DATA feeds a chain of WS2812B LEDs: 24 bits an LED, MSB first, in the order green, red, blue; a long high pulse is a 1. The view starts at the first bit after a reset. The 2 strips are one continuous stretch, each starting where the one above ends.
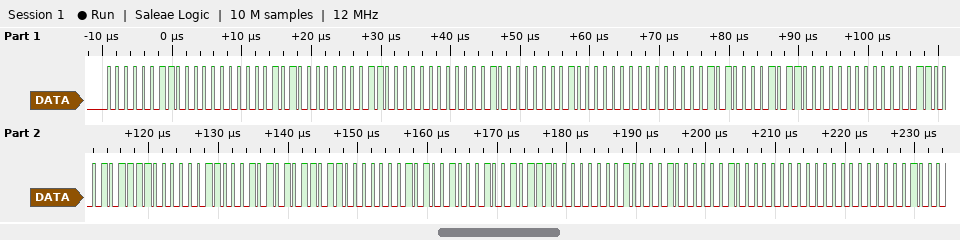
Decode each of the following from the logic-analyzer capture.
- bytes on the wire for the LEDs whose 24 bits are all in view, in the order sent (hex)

03 00 14 03 00 08 04 00 05 0B 00 06 2F 03 15 6C 05 22 5C 02 10 20 00 01
